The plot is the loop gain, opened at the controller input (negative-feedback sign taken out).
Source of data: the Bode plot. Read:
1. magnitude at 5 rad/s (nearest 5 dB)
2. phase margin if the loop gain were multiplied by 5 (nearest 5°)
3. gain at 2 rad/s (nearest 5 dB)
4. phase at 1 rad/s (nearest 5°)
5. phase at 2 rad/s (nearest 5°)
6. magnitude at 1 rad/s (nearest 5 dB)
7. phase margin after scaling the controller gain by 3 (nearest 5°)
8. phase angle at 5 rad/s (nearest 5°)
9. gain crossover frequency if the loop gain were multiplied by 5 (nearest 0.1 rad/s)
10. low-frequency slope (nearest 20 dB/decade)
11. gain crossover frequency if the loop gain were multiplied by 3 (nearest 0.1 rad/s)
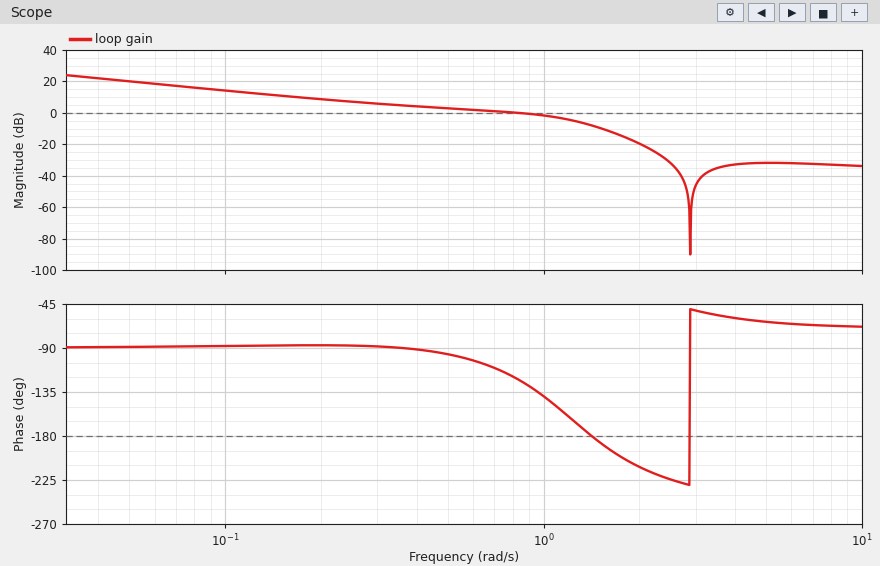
-30 dB
-20°
-20 dB
-140°
-210°
0 dB
-5°
-65°
1.7 rad/s
-20 dB/decade
1.5 rad/s
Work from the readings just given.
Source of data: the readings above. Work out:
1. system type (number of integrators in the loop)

1
